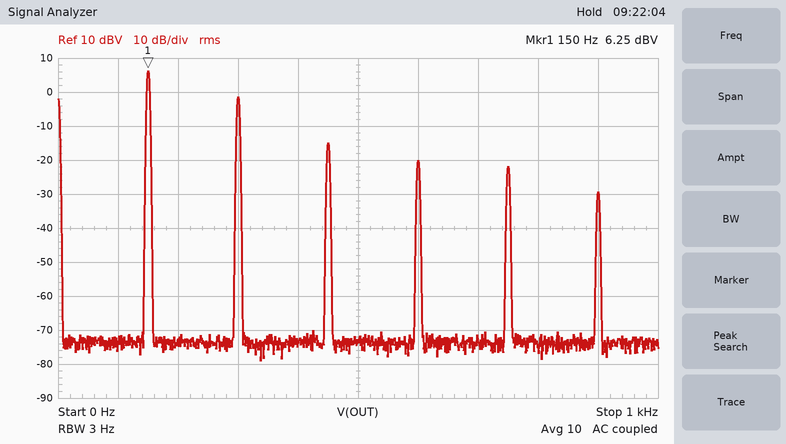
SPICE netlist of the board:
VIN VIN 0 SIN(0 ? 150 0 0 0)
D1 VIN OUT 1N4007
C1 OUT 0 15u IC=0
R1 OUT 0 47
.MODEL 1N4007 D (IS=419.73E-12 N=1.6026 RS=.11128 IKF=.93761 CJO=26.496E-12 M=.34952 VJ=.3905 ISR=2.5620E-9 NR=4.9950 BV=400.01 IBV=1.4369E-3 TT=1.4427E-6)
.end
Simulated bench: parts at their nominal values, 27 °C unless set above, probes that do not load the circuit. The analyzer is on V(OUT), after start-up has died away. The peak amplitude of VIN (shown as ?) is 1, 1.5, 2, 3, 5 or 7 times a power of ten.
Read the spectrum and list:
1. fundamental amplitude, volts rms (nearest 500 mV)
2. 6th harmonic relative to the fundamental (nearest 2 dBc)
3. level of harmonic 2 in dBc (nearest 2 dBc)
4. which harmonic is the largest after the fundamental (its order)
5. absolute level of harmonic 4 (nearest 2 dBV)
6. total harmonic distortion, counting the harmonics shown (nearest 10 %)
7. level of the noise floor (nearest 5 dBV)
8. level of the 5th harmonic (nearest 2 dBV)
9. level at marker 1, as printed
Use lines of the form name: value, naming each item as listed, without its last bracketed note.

fundamental amplitude, volts rms: 2.0 V
6th harmonic relative to the fundamental: -36 dBc
level of harmonic 2 in dBc: -8 dBc
which harmonic is the largest after the fundamental: 2
absolute level of harmonic 4: -20 dBV
total harmonic distortion, counting the harmonics shown: 40 %
level of the noise floor: -75 dBV
level of the 5th harmonic: -22 dBV
level at marker 1, as printed: 6.25 dBV
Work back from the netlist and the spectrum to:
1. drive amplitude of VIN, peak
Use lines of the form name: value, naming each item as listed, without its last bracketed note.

drive amplitude of VIN, peak: 7 V
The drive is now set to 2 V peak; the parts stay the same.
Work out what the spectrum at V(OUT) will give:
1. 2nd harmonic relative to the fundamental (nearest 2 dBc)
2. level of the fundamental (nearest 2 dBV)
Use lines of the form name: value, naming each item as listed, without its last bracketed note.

2nd harmonic relative to the fundamental: -6 dBc
level of the fundamental: -8 dBV
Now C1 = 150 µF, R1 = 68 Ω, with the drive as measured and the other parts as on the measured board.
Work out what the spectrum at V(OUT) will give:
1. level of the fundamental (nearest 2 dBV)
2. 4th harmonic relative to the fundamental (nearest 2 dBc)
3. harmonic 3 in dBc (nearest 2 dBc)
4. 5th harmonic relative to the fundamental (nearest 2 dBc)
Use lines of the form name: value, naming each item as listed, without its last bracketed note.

level of the fundamental: -4 dBV
4th harmonic relative to the fundamental: -16 dBc
harmonic 3 in dBc: -12 dBc
5th harmonic relative to the fundamental: -20 dBc
